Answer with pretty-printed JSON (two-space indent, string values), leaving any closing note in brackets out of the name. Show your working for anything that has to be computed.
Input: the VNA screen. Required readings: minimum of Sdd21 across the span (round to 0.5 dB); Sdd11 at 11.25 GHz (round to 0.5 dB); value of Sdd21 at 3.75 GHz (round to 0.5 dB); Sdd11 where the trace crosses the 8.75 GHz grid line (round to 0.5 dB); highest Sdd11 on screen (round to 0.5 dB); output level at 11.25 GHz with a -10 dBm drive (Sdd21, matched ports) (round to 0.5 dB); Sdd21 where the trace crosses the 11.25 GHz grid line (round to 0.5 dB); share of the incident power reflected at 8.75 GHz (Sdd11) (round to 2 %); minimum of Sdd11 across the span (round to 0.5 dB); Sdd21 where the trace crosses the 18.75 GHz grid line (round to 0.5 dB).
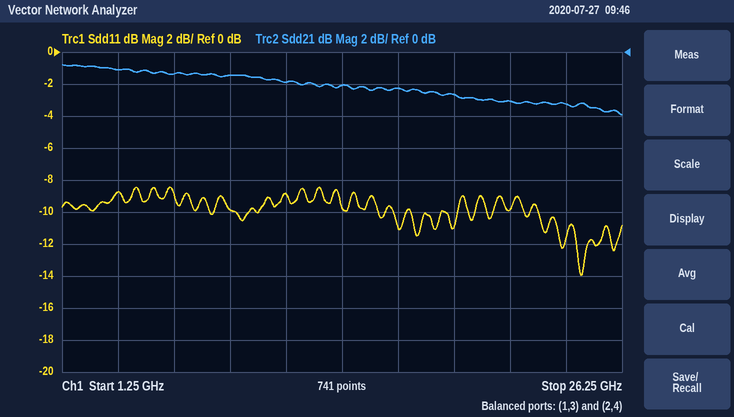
{
  "minimum of Sdd21 across the span": "-4.0 dB",
  "Sdd11 at 11.25 GHz": "-9.0 dB",
  "value of Sdd21 at 3.75 GHz": "-1.0 dB",
  "Sdd11 where the trace crosses the 8.75 GHz grid line": "-10.0 dB",
  "highest Sdd11 on screen": "-8.5 dB",
  "output level at 11.25 GHz with a -10 dBm drive (Sdd21, matched ports)": "-10 dBm + (-2.0 dB) = -12.0 dBm",
  "Sdd21 where the trace crosses the 11.25 GHz grid line": "-2.0 dB",
  "share of the incident power reflected at 8.75 GHz (Sdd11)": "10^(-10/10) ≈ 10 %",
  "minimum of Sdd11 across the span": "-14.0 dB",
  "Sdd21 where the trace crosses the 18.75 GHz grid line": "-2.5 dB"
}
